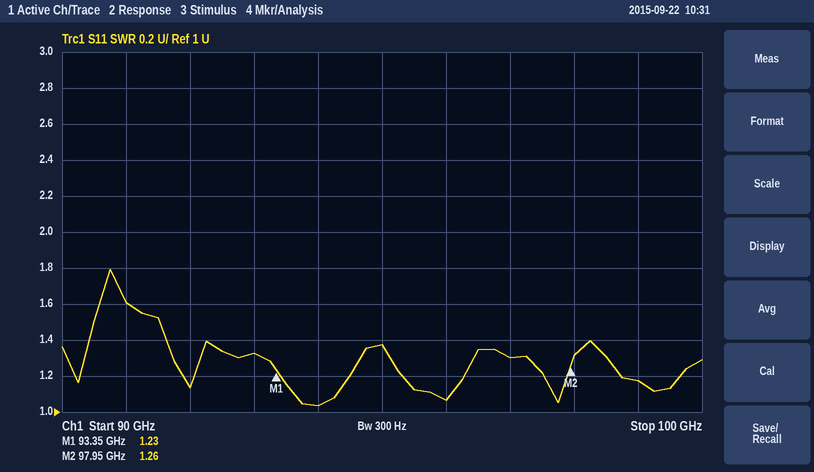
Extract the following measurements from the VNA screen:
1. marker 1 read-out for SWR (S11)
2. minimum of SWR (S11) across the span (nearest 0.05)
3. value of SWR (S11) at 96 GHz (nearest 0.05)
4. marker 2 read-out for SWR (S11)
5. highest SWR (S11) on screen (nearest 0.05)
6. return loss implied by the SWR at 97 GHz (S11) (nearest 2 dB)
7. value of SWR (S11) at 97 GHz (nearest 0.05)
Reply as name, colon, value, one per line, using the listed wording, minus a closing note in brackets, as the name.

marker 1 read-out for SWR: 1.23
minimum of SWR (S11) across the span: 1.05
value of SWR (S11) at 96 GHz: 1.05
marker 2 read-out for SWR: 1.26
highest SWR (S11) on screen: 1.80
return loss implied by the SWR at 97 GHz (S11): 18 dB
value of SWR (S11) at 97 GHz: 1.30
